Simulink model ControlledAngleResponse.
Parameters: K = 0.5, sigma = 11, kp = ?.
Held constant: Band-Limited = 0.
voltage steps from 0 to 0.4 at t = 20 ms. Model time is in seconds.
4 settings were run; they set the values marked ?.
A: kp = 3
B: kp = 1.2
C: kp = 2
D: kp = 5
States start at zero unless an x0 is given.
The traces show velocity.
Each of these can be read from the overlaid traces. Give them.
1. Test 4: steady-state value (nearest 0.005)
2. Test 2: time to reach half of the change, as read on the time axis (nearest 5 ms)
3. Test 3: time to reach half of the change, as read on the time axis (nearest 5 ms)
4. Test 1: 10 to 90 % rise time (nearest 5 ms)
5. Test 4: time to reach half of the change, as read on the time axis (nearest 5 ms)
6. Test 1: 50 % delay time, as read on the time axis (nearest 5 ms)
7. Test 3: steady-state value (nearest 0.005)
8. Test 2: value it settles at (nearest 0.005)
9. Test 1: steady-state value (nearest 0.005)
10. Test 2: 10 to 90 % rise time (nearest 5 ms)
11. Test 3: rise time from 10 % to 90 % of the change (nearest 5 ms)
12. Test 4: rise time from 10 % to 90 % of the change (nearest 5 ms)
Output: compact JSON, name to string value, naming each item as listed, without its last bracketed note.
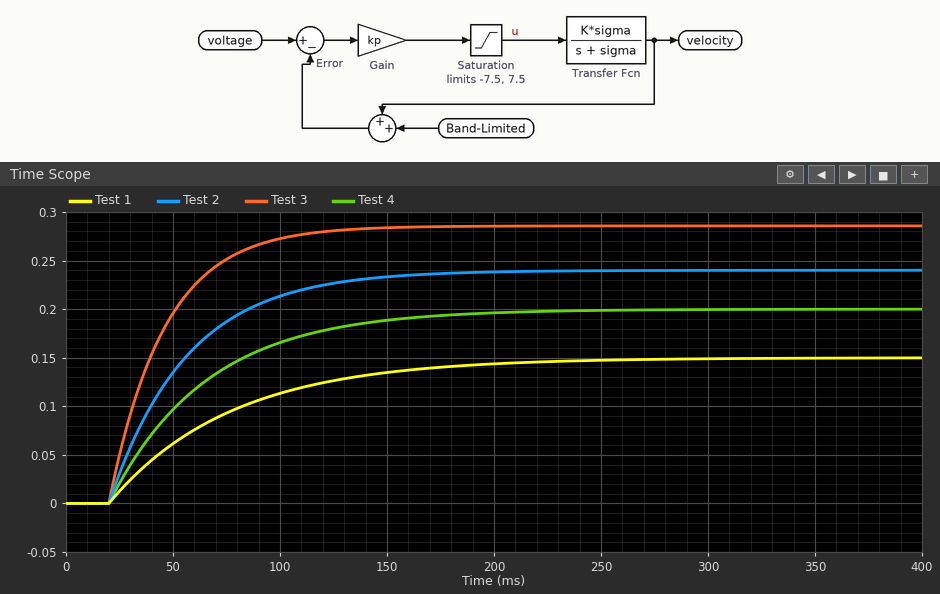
{"Test 4: steady-state value": "0.200", "Test 2: time to reach half of the change, as read on the time axis": "45 ms", "Test 3: time to reach half of the change, as read on the time axis": "40 ms", "Test 1: 10 to 90 % rise time": "125 ms", "Test 4: time to reach half of the change, as read on the time axis": "50 ms", "Test 1: 50 % delay time, as read on the time axis": "60 ms", "Test 3: steady-state value": "0.285", "Test 2: value it settles at": "0.240", "Test 1: steady-state value": "0.150", "Test 2: 10 to 90 % rise time": "80 ms", "Test 3: rise time from 10 % to 90 % of the change": "55 ms", "Test 4: rise time from 10 % to 90 % of the change": "100 ms"}
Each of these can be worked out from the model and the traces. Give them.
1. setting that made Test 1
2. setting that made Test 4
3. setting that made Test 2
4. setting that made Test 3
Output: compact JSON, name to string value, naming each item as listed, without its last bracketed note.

{"setting that made Test 1": "B", "setting that made Test 4": "C", "setting that made Test 2": "A", "setting that made Test 3": "D"}
